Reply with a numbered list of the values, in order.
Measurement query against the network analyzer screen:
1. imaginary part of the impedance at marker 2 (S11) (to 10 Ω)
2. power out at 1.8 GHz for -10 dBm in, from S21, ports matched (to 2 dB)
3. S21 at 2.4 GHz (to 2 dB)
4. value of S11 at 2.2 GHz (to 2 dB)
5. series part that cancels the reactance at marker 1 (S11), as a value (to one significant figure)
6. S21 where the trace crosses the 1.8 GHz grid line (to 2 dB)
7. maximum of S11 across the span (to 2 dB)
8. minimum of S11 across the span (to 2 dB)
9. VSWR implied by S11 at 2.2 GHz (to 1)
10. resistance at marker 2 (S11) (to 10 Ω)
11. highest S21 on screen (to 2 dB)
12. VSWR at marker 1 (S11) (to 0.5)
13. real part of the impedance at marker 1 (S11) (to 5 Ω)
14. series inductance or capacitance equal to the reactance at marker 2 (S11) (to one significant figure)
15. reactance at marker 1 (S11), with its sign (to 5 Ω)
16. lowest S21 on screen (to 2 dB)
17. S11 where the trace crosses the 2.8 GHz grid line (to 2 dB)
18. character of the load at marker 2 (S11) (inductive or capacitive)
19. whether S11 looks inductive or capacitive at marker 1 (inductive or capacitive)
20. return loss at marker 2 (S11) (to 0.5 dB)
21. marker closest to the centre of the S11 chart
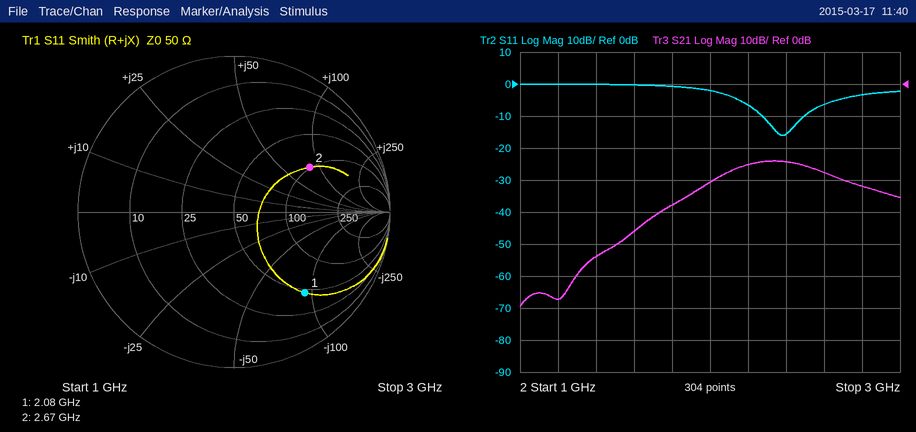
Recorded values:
1. +80 Ω
2. -48 dBm
3. -24 dB
4. -6 dB
5. 7 nH
6. -38 dB
7. 0 dB
8. -16 dB
9. 3
10. 100 Ω
11. -24 dB
12. 5.5
13. 45 Ω
14. 5 nH
15. -90 Ω
16. -70 dB
17. -4 dB
18. inductive
19. capacitive
20. 5.0 dB
21. marker 2
